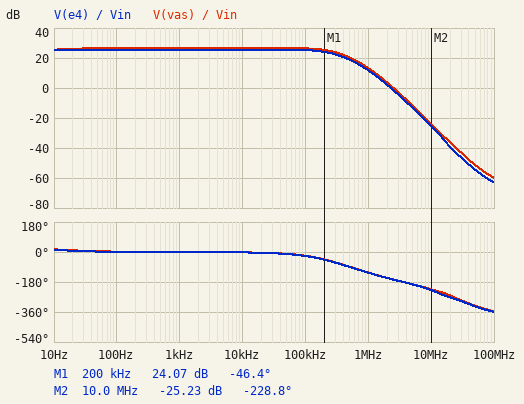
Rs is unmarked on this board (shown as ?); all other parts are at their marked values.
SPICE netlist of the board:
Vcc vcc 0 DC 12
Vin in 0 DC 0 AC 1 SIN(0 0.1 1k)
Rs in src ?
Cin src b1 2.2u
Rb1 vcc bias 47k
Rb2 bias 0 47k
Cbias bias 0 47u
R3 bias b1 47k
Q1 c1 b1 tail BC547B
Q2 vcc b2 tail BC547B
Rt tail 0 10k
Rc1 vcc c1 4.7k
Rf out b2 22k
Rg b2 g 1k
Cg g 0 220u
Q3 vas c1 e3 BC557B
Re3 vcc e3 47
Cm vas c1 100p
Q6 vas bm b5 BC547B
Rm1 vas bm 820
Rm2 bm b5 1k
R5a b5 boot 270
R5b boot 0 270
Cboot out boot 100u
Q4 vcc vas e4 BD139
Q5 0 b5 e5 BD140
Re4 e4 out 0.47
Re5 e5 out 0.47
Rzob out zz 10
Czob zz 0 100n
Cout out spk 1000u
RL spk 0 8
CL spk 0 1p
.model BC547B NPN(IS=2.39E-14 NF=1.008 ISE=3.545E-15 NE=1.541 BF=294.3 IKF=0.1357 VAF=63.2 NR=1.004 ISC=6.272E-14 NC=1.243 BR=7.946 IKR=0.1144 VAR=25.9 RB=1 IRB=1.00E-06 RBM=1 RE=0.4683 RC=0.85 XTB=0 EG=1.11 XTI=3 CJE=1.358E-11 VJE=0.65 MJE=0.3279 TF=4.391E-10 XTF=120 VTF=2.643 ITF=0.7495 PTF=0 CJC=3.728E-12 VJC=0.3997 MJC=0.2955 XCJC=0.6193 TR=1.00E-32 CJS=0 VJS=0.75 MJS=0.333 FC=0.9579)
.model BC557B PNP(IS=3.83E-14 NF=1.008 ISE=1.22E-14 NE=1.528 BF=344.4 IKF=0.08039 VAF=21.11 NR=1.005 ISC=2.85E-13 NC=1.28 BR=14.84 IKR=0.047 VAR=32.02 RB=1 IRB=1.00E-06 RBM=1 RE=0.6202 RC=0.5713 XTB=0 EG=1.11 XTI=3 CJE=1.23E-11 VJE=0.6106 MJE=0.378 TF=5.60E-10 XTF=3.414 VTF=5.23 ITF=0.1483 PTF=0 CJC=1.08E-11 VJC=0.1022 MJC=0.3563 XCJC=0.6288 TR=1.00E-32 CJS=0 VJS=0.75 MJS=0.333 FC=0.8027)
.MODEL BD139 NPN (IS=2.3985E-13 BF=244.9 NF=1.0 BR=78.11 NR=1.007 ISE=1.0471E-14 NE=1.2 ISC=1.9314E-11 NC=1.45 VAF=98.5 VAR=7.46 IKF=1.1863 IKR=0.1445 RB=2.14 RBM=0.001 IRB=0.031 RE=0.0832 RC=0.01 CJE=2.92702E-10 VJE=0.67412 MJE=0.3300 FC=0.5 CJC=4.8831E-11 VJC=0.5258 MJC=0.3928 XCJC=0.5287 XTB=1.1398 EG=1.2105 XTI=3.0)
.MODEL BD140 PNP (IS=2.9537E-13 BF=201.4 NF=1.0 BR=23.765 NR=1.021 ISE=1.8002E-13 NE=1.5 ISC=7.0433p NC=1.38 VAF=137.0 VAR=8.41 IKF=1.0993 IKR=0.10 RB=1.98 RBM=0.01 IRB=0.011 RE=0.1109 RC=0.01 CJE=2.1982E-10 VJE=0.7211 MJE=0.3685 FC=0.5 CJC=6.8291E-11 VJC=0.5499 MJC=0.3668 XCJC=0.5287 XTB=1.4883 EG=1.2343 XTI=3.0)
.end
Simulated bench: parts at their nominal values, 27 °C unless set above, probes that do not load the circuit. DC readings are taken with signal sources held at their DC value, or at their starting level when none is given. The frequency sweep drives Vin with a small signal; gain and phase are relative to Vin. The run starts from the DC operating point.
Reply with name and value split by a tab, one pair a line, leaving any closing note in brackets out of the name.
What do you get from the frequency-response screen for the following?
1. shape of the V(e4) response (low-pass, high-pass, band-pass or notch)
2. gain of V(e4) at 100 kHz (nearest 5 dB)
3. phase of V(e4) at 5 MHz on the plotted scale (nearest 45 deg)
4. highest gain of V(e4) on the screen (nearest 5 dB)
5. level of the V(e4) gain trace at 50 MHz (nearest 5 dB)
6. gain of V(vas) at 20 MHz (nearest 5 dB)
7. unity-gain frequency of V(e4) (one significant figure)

shape of the V(e4) response	low-pass
gain of V(e4) at 100 kHz	25 dB
phase of V(e4) at 5 MHz on the plotted scale	-180 deg
highest gain of V(e4) on the screen	25 dB
level of the V(e4) gain trace at 50 MHz	-55 dB
gain of V(vas) at 20 MHz	-35 dB
unity-gain frequency of V(e4)	2 MHz
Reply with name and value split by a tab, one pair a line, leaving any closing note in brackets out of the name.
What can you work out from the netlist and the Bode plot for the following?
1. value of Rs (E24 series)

value of Rs	6.8 kΩ
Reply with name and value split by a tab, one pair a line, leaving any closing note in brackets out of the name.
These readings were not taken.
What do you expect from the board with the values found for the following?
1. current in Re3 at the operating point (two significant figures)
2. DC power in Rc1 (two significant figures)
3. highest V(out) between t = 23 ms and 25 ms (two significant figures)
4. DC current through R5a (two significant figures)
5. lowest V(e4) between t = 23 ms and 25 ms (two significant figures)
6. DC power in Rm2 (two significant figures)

current in Re3 at the operating point	9.8 mA
DC power in Rc1	280 µW
highest V(out) between t = 23 ms and 25 ms	7.8 V
DC current through R5a	9.8 mA
lowest V(e4) between t = 23 ms and 25 ms	4.1 V
DC power in Rm2	490 µW
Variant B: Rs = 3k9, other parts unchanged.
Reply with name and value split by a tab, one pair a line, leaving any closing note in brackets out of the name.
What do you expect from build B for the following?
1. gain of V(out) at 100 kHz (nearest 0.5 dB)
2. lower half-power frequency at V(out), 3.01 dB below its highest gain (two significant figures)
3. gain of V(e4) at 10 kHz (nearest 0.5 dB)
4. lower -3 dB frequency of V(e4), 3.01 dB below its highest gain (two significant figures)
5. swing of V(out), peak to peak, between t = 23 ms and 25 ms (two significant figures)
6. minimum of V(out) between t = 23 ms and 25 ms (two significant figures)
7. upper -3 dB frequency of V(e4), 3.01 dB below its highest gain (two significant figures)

gain of V(out) at 100 kHz	25.5 dB
lower half-power frequency at V(out), 3.01 dB below its highest gain	2.0 Hz
gain of V(e4) at 10 kHz	26.0 dB
lower -3 dB frequency of V(e4), 3.01 dB below its highest gain	2.1 Hz
swing of V(out), peak to peak, between t = 23 ms and 25 ms	3.9 V
minimum of V(out) between t = 23 ms and 25 ms	4.0 V
upper -3 dB frequency of V(e4), 3.01 dB below its highest gain	290 kHz
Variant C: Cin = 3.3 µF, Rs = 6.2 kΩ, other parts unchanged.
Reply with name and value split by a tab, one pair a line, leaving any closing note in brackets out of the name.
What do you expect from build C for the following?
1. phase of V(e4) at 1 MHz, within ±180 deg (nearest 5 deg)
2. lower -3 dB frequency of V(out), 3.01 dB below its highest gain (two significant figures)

phase of V(e4) at 1 MHz, within ±180 deg	-120 deg
lower -3 dB frequency of V(out), 3.01 dB below its highest gain	1.5 Hz
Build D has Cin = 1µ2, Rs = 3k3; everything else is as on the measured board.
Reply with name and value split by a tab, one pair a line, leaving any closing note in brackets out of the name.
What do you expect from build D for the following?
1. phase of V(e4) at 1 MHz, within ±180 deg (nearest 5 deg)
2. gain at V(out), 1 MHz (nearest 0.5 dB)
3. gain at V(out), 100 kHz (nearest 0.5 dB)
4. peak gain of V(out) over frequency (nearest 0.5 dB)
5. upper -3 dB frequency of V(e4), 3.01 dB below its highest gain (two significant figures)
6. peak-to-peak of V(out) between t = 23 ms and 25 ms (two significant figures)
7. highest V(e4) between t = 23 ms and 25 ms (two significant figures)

phase of V(e4) at 1 MHz, within ±180 deg	-110 deg
gain at V(out), 1 MHz	13.5 dB
gain at V(out), 100 kHz	25.5 dB
peak gain of V(out) over frequency	26.0 dB
upper -3 dB frequency of V(e4), 3.01 dB below its highest gain	290 kHz
peak-to-peak of V(out) between t = 23 ms and 25 ms	4.0 V
highest V(e4) between t = 23 ms and 25 ms	8.1 V
